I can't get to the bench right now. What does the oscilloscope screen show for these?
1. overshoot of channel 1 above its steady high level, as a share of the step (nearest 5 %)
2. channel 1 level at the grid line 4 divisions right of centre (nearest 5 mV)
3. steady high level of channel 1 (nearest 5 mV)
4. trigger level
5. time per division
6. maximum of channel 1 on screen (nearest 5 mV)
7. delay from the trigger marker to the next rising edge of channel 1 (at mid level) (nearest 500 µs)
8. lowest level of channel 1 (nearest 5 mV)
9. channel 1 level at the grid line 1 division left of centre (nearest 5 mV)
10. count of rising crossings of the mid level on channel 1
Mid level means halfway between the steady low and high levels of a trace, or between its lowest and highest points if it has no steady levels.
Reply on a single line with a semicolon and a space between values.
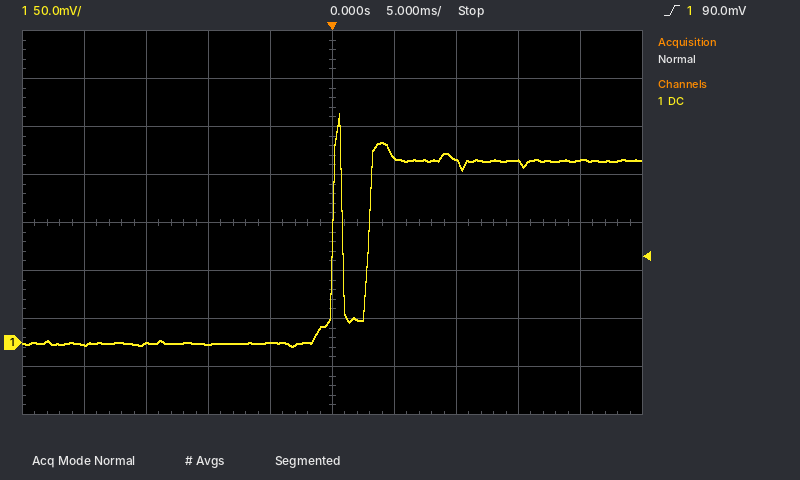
25 %; 190 mV; 190 mV; 90.0 mV; 5 ms; 240 mV; 3.0 ms; -5 mV; 0 mV; 2
